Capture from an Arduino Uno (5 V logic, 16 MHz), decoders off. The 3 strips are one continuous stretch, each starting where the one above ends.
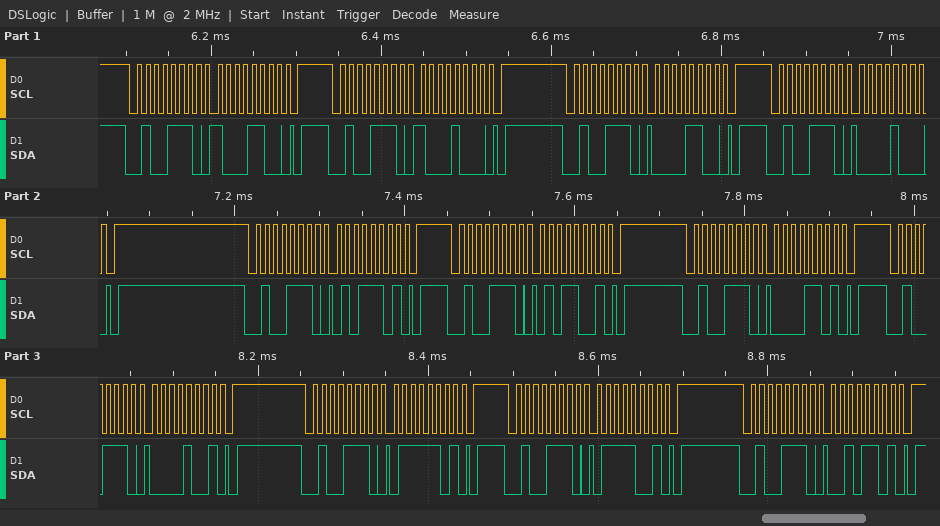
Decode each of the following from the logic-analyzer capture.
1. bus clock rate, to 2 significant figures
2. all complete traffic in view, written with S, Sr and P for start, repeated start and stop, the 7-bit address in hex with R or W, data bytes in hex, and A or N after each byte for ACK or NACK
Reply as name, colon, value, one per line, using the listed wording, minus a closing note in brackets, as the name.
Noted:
bus clock rate, to 2 significant figures: 100 kHz
all complete traffic in view, written with S, Sr and P for start, repeated start and stop, the 7-bit address in hex with R or W, data bytes in hex, and A or N after each byte for ACK or NACK: S 27W A 8C A P S 27W A 88 A P S 27W A 0C A P S 27W A 08 A P S 27W A 5D A P S 27W A 59 A P S 27W A 0D A P S 27W A 09 A P S 27W A 7D A P S 27W A 79 A P S 27W A 2D A P
